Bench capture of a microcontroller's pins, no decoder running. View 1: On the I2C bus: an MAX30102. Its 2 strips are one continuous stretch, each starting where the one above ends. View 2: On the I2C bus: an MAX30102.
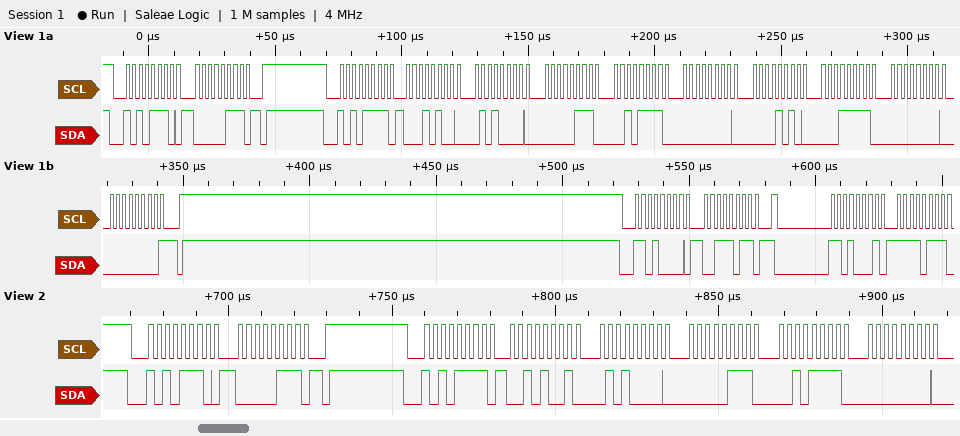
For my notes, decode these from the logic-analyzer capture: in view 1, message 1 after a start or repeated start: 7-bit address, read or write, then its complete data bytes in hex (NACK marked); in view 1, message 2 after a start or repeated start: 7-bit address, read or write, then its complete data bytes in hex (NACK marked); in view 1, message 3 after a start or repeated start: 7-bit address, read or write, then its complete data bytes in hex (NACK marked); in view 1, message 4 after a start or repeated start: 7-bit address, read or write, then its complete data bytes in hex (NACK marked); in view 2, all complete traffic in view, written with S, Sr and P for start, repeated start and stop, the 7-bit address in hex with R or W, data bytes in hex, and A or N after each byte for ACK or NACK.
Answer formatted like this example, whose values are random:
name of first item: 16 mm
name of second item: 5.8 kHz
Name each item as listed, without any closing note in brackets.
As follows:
in view 1, message 1 after a start or repeated start: 7-bit address, read or write, then its complete data bytes in hex: 0x57 write: 07
in view 1, message 2 after a start or repeated start: 7-bit address, read or write, then its complete data bytes in hex: 0x57 read: 14 50 07 2F 00 0A 1F 00 00 NACK
in view 1, message 3 after a start or repeated start: 7-bit address, read or write, then its complete data bytes in hex: 0x68 write: 3B
in view 1, message 4 after a start or repeated start: 7-bit address, read or write, then its complete data bytes in hex: 0x68 read: F7
in view 2, all complete traffic in view, written with S, Sr and P for start, repeated start and stop, the 7-bit address in hex with R or W, data bytes in hex, and A or N after each byte for ACK or NACK: S 57W A 07 A P S 57R A 29 A 50 A 07 A 2F A 00 A
